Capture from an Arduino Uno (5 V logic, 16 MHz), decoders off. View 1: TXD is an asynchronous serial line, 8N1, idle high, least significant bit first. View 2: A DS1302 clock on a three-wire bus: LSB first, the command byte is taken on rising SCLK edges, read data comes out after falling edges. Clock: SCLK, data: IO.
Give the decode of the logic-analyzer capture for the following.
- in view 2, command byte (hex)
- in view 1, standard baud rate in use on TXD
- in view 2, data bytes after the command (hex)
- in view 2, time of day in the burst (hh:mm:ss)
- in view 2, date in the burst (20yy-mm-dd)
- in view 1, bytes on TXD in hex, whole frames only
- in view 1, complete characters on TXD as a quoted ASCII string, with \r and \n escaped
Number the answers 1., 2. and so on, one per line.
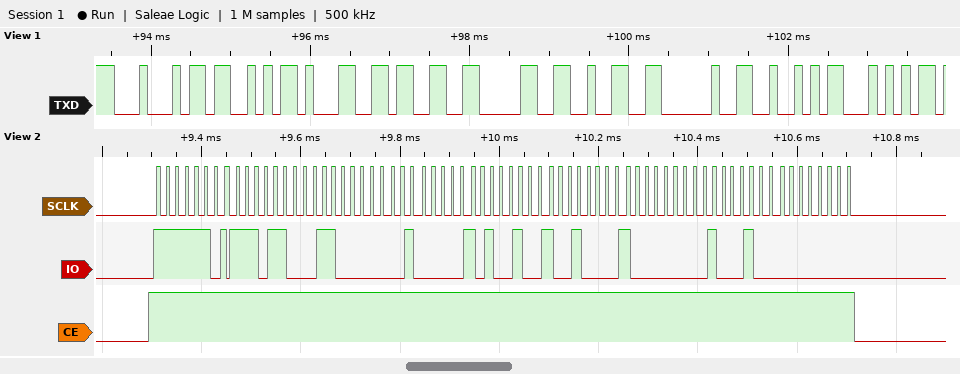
1. 0xBF
2. 9600 baud
3. 37 06 04 25 09 01 22 00
4. 04:06:37
5. 2022-09-25
6. 44 53 31 33 30 32 20 52 54
7. "DS1302 RT"
